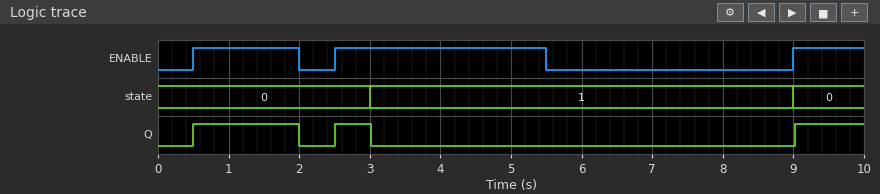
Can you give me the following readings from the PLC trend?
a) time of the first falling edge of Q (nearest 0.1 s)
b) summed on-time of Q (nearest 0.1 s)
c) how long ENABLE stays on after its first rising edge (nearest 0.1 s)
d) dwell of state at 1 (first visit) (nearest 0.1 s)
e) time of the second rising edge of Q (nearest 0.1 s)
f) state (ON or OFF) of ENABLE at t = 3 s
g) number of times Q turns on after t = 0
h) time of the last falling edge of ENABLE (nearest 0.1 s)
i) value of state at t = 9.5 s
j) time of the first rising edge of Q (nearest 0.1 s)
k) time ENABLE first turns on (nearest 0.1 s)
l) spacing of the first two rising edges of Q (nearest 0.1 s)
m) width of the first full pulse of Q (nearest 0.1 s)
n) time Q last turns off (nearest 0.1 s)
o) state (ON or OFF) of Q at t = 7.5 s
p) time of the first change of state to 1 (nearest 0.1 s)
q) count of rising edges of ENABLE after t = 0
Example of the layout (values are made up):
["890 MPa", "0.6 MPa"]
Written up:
["2.0 s", "3.0 s", "1.5 s", "6.0 s", "2.5 s", "ON", "3", "5.5 s", "0", "0.5 s", "0.5 s", "2.0 s", "1.5 s", "3.0 s", "OFF", "3.0 s", "3"]
